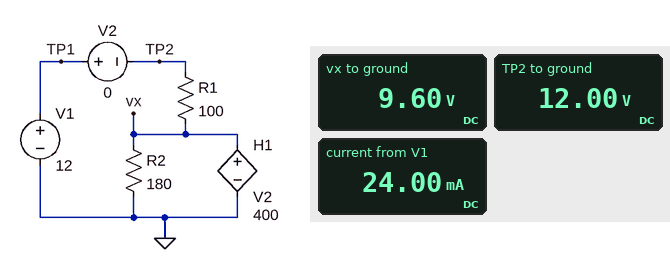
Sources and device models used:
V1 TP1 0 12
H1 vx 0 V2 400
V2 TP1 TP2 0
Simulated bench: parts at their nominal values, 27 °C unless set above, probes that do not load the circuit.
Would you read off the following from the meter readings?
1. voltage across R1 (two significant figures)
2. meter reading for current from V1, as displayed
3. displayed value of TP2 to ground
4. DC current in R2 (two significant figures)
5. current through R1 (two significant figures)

2.4 V
24.00 mA
12.00 V
53 mA
24 mA
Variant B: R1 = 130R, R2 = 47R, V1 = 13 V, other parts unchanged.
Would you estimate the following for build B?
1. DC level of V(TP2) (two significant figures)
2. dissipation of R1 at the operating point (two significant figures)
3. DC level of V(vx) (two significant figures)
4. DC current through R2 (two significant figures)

13 V
78 mW
9.8 V
210 mA
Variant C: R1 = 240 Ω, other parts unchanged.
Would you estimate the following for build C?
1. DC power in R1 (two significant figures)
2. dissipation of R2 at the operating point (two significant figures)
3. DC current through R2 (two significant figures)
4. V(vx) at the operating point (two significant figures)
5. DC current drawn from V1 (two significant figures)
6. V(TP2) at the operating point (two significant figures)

84 mW
310 mW
42 mA
7.5 V
19 mA
12 V
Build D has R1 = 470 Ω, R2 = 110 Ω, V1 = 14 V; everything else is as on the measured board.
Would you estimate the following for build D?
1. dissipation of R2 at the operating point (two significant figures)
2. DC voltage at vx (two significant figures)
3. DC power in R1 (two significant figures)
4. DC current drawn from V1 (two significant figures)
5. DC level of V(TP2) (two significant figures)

380 mW
6.4 V
120 mW
16 mA
14 V
